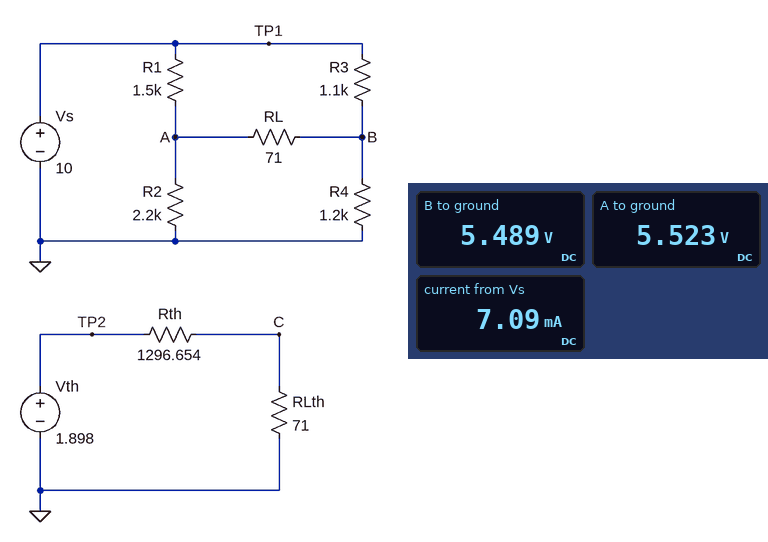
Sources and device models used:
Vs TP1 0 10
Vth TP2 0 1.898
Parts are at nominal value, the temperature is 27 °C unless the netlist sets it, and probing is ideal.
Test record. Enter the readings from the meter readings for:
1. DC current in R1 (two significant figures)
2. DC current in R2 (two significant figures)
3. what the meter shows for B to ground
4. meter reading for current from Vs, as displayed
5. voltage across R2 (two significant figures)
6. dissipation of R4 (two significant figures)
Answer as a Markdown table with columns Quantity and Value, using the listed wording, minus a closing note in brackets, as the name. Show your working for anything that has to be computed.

| Quantity | Value |
|---|---|
| DC current in R1 | (10 V - 5.523 V) / 1.5 kΩ = 3.0 mA |
| DC current in R2 | (5.523 V) / 2.2 kΩ = 2.5 mA |
| what the meter shows for B to ground | 5.489 V |
| meter reading for current from Vs, as displayed | 7.09 mA |
| voltage across R2 | 5.523 V = 5.5 V |
| dissipation of R4 | (5.489 V)^2 / 1.2 kΩ = 25 mW |
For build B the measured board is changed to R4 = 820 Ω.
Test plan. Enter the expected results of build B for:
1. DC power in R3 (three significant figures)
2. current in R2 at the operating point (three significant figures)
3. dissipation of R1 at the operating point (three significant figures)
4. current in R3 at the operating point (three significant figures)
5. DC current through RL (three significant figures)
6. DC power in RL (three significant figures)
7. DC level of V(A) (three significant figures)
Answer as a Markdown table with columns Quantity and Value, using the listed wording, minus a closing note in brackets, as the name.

| Quantity | Value |
|---|---|
| DC power in R3 | 24.4 mW |
| current in R2 at the operating point | 2.23 mA |
| dissipation of R1 at the operating point | 17.3 mW |
| current in R3 at the operating point | 4.71 mA |
| DC current through RL | 1.17 mA |
| DC power in RL | 97.1 µW |
| DC level of V(A) | 4.90 V |
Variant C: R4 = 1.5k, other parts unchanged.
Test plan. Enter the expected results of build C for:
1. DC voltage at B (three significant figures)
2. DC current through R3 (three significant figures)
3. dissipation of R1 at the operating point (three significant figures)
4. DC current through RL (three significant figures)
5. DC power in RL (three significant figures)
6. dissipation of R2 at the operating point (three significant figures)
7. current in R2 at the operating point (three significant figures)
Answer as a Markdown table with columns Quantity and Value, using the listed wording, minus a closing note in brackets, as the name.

| Quantity | Value |
|---|---|
| DC voltage at B | 5.84 V |
| DC current through R3 | 3.78 mA |
| dissipation of R1 at the operating point | 11.5 mW |
| DC current through RL | 111 µA |
| DC power in RL | 869 nW |
| dissipation of R2 at the operating point | 15.5 mW |
| current in R2 at the operating point | 2.66 mA |
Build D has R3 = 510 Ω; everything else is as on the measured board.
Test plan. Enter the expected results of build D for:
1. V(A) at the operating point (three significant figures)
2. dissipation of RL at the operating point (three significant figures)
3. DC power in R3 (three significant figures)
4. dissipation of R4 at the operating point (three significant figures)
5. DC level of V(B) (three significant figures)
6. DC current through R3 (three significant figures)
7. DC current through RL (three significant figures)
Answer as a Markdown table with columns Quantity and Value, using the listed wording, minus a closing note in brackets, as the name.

| Quantity | Value |
|---|---|
| V(A) at the operating point | 6.67 V |
| dissipation of RL at the operating point | 46.7 µW |
| DC power in R3 | 21.0 mW |
| dissipation of R4 at the operating point | 37.7 mW |
| DC level of V(B) | 6.73 V |
| DC current through R3 | 6.42 mA |
| DC current through RL | 811 µA |
